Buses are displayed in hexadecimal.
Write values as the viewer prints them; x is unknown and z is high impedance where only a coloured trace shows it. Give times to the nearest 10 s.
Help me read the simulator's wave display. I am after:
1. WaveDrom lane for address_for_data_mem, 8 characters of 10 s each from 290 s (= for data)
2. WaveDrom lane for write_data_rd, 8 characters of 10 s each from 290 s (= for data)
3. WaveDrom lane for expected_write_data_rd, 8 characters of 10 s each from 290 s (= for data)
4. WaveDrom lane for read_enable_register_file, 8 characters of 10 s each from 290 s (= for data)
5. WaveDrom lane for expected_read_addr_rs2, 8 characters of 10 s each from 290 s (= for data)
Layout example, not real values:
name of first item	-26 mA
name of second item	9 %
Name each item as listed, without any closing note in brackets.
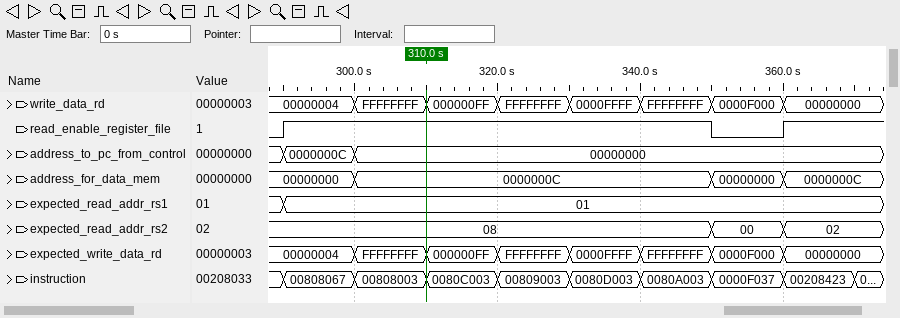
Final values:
WaveDrom lane for address_for_data_mem, 8 characters of 10 s each from 290 s	{name: 'address_for_data_mem', wave: '==....==', data: '00000000 0000000C 00000000 0000000C'}
WaveDrom lane for write_data_rd, 8 characters of 10 s each from 290 s	{name: 'write_data_rd', wave: '========', data: '00000004 FFFFFFFF 000000FF FFFFFFFF 0000FFFF FFFFFFFF 0000F000 00000000'}
WaveDrom lane for expected_write_data_rd, 8 characters of 10 s each from 290 s	{name: 'expected_write_data_rd', wave: '========', data: '00000004 FFFFFFFF 000000FF FFFFFFFF 0000FFFF FFFFFFFF 0000F000 00000000'}
WaveDrom lane for read_enable_register_file, 8 characters of 10 s each from 290 s	{name: 'read_enable_register_file', wave: '1.....01'}
WaveDrom lane for expected_read_addr_rs2, 8 characters of 10 s each from 290 s	{name: 'expected_read_addr_rs2', wave: '=.....==', data: '08 00 02'}
